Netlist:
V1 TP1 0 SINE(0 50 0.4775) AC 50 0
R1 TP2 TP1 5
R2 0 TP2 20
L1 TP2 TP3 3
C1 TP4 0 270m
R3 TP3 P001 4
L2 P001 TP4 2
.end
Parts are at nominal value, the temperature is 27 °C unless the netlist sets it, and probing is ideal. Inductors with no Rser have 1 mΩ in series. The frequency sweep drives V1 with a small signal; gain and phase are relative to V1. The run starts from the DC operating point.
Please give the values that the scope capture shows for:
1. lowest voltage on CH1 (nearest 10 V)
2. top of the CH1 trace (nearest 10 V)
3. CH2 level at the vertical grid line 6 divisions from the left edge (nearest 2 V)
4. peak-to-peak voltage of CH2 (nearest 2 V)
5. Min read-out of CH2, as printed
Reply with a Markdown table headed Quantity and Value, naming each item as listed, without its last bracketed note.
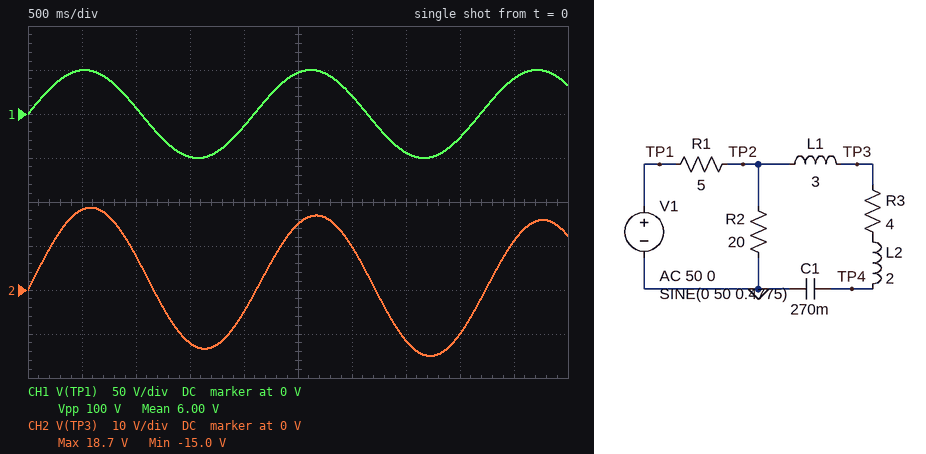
| Quantity | Value |
|---|---|
| lowest voltage on CH1 | -50 V |
| top of the CH1 trace | 50 V |
| CH2 level at the vertical grid line 6 divisions from the left edge | 10 V |
| peak-to-peak voltage of CH2 | 34 V |
| Min read-out of CH2, as printed | -15.0 V |
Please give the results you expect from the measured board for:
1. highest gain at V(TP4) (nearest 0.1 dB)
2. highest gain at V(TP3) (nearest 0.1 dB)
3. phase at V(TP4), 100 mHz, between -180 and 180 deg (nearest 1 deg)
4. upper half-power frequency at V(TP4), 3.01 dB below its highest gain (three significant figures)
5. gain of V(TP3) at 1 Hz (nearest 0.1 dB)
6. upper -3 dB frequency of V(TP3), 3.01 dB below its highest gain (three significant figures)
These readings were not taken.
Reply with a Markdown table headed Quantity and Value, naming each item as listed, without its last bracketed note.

| Quantity | Value |
|---|---|
| highest gain at V(TP4) | -1.9 dB |
| highest gain at V(TP3) | -1.9 dB |
| phase at V(TP4), 100 mHz, between -180 and 180 deg | -71 deg |
| upper half-power frequency at V(TP4), 3.01 dB below its highest gain | 97.7 mHz |
| gain of V(TP3) at 1 Hz | -10.0 dB |
| upper -3 dB frequency of V(TP3), 3.01 dB below its highest gain | 104 mHz |
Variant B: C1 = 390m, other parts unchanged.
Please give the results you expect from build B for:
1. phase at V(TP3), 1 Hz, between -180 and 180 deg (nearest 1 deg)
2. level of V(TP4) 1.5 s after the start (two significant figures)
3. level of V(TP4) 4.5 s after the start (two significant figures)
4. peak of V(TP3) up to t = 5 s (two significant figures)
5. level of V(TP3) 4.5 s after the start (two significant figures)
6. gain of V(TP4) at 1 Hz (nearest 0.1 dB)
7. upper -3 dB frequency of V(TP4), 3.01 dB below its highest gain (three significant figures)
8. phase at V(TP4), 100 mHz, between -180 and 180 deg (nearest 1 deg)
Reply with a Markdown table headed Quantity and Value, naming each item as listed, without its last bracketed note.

| Quantity | Value |
|---|---|
| phase at V(TP3), 1 Hz, between -180 and 180 deg | -4 deg |
| level of V(TP4) 1.5 s after the start | 5.4 V |
| level of V(TP4) 4.5 s after the start | -860 mV |
| peak of V(TP3) up to t = 5 s | 18 V |
| level of V(TP3) 4.5 s after the start | 12 V |
| gain of V(TP4) at 1 Hz | -39.8 dB |
| upper -3 dB frequency of V(TP4), 3.01 dB below its highest gain | 62.8 mHz |
| phase at V(TP4), 100 mHz, between -180 and 180 deg | -83 deg |
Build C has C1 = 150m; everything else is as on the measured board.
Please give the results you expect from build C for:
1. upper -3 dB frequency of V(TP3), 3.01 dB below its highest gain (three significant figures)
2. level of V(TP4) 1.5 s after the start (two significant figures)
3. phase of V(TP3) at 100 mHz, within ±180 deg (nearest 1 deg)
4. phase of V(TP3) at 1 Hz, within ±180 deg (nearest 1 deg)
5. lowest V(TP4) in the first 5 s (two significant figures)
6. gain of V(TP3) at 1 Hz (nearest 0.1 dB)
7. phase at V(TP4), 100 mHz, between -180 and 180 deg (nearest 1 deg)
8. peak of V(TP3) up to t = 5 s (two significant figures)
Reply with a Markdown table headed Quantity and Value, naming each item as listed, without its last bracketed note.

| Quantity | Value |
|---|---|
| upper -3 dB frequency of V(TP3), 3.01 dB below its highest gain | 171 mHz |
| level of V(TP4) 1.5 s after the start | 12 V |
| phase of V(TP3) at 100 mHz, within ±180 deg | -24 deg |
| phase of V(TP3) at 1 Hz, within ±180 deg | -4 deg |
| lowest V(TP4) in the first 5 s | -6.3 V |
| gain of V(TP3) at 1 Hz | -10.2 dB |
| phase at V(TP4), 100 mHz, between -180 and 180 deg | -47 deg |
| peak of V(TP3) up to t = 5 s | 20 V |
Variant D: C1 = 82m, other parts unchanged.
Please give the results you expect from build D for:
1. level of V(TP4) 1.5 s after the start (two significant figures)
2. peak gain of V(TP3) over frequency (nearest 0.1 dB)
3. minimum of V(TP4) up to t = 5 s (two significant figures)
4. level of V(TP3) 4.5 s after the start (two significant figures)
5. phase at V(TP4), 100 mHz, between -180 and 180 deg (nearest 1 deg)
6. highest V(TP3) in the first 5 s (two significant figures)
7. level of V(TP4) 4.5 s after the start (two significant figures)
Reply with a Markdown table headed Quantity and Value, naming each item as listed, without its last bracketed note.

| Quantity | Value |
|---|---|
| level of V(TP4) 1.5 s after the start | 17 V |
| peak gain of V(TP3) over frequency | -1.7 dB |
| minimum of V(TP4) up to t = 5 s | -13 V |
| level of V(TP3) 4.5 s after the start | 5.7 V |
| phase at V(TP4), 100 mHz, between -180 and 180 deg | -26 deg |
| highest V(TP3) in the first 5 s | 22 V |
| level of V(TP4) 4.5 s after the start | -12 V |
